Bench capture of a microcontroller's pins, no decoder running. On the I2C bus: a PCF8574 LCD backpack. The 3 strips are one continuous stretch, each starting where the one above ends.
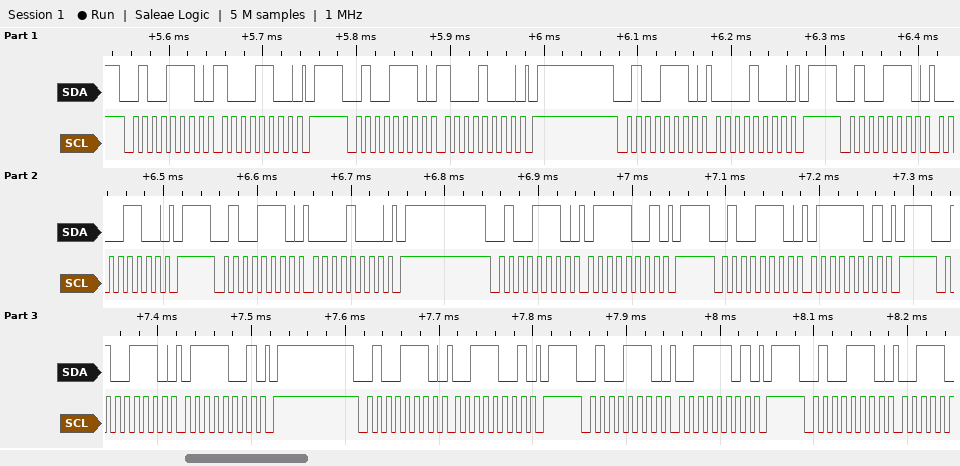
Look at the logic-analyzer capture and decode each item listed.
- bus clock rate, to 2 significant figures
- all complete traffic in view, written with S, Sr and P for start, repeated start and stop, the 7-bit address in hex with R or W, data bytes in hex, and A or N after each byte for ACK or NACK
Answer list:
100 kHz
S 27W A 8C A P S 27W A 88 A P S 27W A 08 A P S 27W A 0C A P S 27W A 08 A P S 27W A 79 A P S 27W A 7D A P S 27W A 79 A P S 27W A 39 A P S 27W A 3D A P S 27W A
